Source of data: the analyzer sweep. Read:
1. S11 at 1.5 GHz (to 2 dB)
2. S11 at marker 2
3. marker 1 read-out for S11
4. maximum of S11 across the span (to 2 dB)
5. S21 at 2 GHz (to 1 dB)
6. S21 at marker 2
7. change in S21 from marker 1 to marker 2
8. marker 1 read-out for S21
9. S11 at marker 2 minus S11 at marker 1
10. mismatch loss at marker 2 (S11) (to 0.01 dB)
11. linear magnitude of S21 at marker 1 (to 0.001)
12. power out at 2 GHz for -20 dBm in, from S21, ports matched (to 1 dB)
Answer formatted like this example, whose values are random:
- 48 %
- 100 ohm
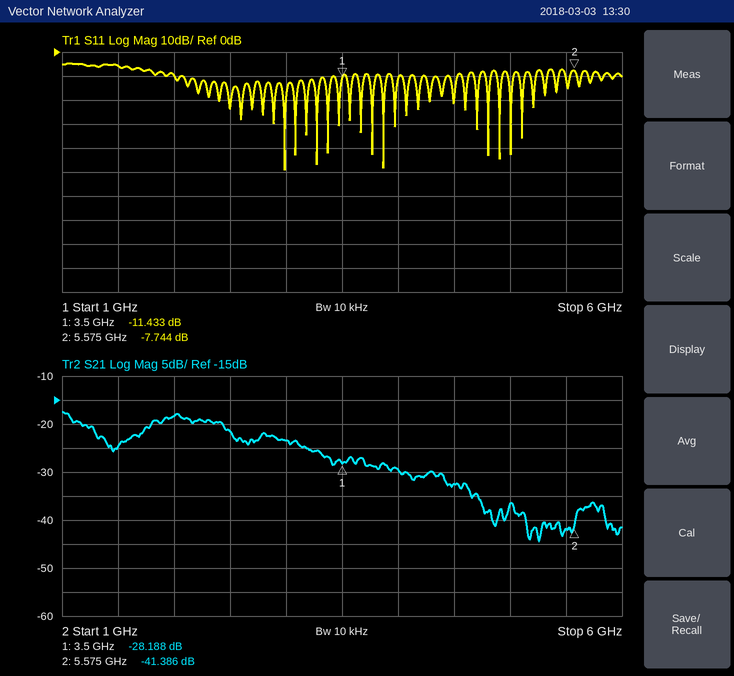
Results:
- -6 dB
- -7.744 dB
- -11.433 dB
- -4 dB
- -18 dB
- -41.386 dB
- -13.198 dB
- -28.188 dB
- 3.689 dB
- 0.80 dB
- 0.039
- -38 dBm
